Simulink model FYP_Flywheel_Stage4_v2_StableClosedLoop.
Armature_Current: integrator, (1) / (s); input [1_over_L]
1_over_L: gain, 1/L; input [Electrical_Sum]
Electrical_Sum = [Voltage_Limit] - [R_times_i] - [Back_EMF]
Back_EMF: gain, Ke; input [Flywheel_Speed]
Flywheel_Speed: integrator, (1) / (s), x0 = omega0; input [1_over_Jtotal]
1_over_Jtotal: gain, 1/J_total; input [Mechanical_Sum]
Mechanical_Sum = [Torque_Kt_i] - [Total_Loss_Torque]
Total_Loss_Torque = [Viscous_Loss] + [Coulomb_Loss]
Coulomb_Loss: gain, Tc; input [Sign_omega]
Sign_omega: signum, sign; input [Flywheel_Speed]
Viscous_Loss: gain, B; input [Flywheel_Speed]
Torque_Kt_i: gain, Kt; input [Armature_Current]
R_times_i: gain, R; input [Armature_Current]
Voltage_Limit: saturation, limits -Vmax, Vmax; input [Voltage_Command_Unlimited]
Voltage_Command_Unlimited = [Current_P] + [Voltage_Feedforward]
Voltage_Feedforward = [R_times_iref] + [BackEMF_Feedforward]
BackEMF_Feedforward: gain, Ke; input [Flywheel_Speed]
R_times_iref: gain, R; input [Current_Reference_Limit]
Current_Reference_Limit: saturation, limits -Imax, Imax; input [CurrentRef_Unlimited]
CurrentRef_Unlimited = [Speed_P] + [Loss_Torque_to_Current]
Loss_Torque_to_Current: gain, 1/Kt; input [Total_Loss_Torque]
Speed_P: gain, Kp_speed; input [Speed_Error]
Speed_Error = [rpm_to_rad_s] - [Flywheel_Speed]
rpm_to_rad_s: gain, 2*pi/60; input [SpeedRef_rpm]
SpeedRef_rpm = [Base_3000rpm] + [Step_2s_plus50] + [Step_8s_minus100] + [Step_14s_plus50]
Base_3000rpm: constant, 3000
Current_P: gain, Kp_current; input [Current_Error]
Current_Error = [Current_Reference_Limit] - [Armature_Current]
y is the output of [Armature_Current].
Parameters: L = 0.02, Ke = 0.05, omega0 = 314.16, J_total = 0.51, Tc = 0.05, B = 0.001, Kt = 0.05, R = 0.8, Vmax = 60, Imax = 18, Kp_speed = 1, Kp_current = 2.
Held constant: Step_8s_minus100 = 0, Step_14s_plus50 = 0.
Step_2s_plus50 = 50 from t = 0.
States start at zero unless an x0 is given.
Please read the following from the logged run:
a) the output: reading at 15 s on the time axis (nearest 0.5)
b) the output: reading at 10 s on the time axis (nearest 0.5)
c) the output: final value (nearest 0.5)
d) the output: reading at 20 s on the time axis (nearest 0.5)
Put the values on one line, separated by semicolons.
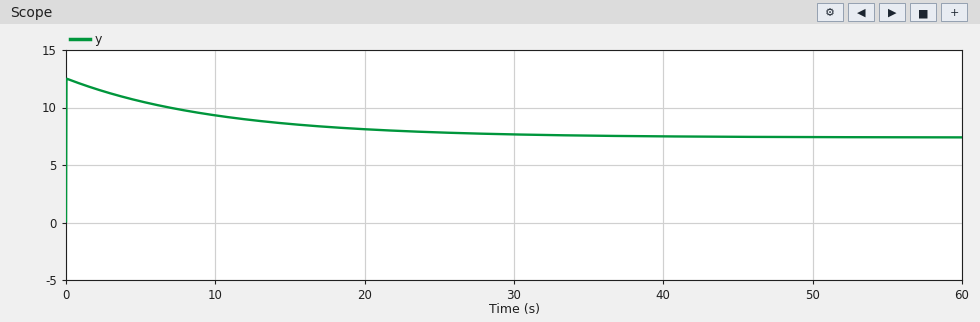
8.5; 9.5; 7.5; 8.0
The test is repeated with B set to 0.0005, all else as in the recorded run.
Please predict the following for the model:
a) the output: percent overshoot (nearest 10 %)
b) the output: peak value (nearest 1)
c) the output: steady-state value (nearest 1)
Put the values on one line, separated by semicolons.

120 %; 9; 4
